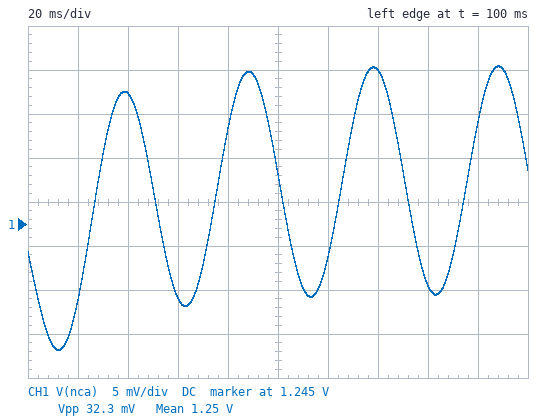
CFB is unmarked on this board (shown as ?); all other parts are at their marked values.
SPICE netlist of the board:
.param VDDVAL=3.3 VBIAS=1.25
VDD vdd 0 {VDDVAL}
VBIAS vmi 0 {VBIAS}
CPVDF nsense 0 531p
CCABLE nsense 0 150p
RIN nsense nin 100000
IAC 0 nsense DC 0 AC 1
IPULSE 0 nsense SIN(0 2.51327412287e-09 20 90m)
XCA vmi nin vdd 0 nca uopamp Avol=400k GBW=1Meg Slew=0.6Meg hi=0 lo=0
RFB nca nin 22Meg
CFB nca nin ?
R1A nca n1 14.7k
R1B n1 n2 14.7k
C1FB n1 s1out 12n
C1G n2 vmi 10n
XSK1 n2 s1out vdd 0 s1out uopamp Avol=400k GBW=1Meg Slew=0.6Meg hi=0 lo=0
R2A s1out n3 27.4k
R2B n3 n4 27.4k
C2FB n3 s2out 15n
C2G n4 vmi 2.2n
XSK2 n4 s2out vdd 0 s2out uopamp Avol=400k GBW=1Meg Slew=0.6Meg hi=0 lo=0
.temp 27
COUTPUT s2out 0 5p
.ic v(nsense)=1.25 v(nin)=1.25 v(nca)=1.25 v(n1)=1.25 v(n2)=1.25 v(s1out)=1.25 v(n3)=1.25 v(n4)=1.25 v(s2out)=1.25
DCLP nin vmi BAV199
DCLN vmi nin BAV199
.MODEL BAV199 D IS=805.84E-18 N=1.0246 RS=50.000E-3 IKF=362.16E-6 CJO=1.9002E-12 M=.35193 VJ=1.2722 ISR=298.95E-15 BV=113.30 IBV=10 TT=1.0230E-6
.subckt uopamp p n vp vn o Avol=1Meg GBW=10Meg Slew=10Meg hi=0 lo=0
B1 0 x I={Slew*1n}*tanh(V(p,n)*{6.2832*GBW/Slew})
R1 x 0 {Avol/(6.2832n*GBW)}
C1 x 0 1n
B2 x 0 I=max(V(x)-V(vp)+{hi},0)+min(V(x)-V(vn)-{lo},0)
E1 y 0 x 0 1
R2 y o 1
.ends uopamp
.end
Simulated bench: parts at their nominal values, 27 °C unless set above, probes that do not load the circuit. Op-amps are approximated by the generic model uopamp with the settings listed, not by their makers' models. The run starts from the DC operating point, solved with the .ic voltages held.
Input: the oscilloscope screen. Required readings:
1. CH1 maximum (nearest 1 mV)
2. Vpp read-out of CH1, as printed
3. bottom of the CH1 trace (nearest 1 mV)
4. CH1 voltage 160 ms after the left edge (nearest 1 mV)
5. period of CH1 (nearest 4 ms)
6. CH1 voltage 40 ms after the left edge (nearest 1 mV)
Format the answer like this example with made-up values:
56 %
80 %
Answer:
1.263 V
32.3 mV
1.231 V
1.238 V
48 ms
1.260 V
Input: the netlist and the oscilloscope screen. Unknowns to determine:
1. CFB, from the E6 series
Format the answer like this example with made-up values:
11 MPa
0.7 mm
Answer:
1.5 nF
